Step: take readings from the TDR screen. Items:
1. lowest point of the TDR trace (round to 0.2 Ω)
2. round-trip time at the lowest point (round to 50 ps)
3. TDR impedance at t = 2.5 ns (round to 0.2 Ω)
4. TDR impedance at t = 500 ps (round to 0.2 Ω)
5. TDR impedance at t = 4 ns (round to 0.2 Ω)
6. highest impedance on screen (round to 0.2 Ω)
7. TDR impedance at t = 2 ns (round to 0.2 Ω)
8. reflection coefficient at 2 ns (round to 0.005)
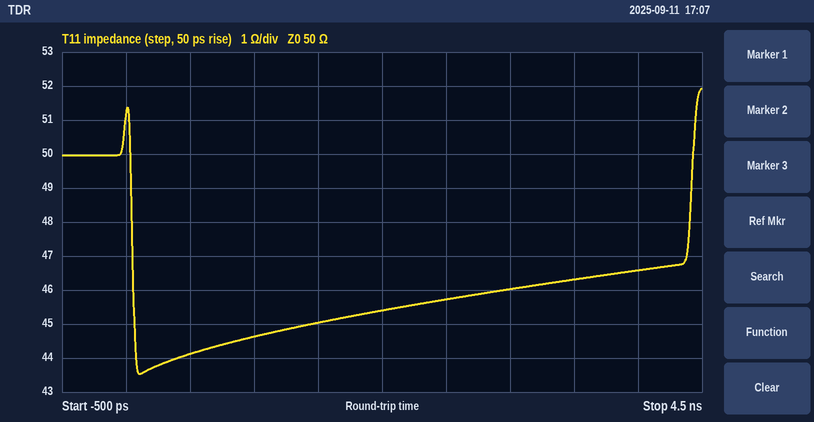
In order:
43.6 Ω
100 ps
45.8 Ω
44.2 Ω
46.6 Ω
52.0 Ω
45.4 Ω
-0.050
